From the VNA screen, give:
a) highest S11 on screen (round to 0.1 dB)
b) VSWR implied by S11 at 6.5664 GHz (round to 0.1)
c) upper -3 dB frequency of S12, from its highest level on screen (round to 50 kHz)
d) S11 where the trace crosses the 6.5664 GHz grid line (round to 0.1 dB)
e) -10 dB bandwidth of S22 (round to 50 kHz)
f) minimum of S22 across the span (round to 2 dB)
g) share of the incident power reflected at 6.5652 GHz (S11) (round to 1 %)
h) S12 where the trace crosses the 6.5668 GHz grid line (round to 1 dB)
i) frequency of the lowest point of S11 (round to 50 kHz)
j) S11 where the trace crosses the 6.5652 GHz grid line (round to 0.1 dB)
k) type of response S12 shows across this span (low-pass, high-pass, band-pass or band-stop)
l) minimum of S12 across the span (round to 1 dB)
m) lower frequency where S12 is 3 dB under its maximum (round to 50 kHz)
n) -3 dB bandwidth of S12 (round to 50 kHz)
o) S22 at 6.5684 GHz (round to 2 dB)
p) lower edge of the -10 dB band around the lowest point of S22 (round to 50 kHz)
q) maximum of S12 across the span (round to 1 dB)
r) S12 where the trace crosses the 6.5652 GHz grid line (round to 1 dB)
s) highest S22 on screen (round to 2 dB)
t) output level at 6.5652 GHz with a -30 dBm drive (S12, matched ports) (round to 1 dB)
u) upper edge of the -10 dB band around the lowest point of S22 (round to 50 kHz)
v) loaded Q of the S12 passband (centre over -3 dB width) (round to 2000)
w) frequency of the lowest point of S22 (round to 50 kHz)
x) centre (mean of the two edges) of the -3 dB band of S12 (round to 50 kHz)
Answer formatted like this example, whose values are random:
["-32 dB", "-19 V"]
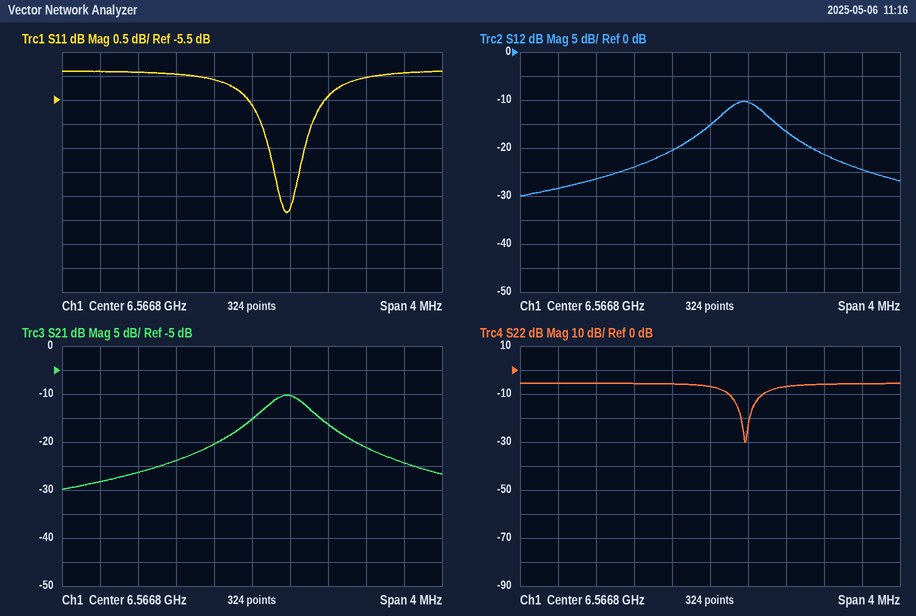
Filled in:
["-4.9 dB", "3.5", "6.56740 GHz", "-5.1 dB", "350 kHz", "-30 dB", "32 %", "-15 dB", "6.56715 GHz", "-4.9 dB", "band-pass", "-30 dB", "6.56690 GHz", "500 kHz", "-6 dB", "6.56700 GHz", "-10 dB", "-28 dB", "-6 dB", "-58 dBm", "6.56735 GHz", "14000", "6.56715 GHz", "6.56715 GHz"]
